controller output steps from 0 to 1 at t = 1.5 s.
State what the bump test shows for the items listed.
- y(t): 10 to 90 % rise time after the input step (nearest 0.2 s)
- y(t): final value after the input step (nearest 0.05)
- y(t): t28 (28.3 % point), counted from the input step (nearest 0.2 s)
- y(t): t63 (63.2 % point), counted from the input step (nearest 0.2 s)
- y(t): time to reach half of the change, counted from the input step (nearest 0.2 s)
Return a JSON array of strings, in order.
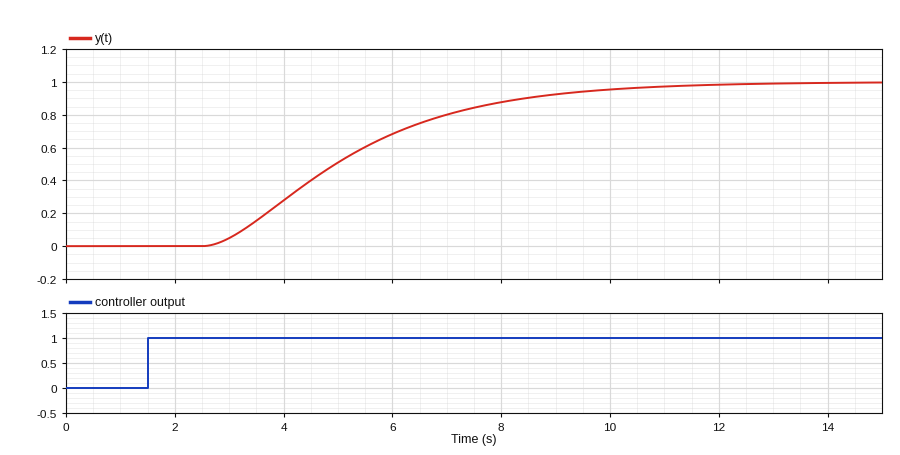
["5.2 s", "1.00", "2.6 s", "4.2 s", "3.4 s"]
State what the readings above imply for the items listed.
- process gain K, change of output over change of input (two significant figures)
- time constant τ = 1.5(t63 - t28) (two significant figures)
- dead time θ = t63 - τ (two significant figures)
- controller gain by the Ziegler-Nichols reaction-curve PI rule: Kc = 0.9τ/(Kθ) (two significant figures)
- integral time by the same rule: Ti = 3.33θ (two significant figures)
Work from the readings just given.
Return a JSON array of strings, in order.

["1.0", "2.4 s", "1.8 s", "1.2", "6.0 s"]
